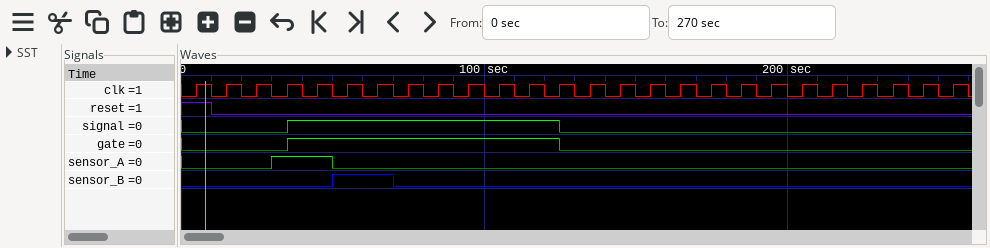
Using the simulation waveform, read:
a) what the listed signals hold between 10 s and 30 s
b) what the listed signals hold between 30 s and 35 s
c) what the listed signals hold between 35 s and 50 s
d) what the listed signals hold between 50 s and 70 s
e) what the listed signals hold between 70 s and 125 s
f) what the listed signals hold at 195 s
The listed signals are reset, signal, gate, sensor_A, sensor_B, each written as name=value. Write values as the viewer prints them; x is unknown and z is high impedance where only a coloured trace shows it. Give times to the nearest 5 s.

reset=0, signal=0, gate=0, sensor_A=0, sensor_B=0
reset=0, signal=0, gate=0, sensor_A=1, sensor_B=0
reset=0, signal=1, gate=1, sensor_A=1, sensor_B=0
reset=0, signal=1, gate=1, sensor_A=0, sensor_B=1
reset=0, signal=1, gate=1, sensor_A=0, sensor_B=0
reset=0, signal=0, gate=0, sensor_A=0, sensor_B=0
